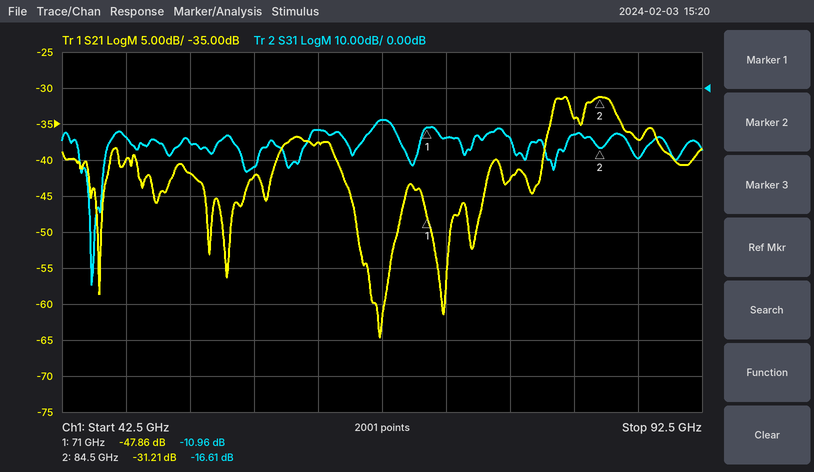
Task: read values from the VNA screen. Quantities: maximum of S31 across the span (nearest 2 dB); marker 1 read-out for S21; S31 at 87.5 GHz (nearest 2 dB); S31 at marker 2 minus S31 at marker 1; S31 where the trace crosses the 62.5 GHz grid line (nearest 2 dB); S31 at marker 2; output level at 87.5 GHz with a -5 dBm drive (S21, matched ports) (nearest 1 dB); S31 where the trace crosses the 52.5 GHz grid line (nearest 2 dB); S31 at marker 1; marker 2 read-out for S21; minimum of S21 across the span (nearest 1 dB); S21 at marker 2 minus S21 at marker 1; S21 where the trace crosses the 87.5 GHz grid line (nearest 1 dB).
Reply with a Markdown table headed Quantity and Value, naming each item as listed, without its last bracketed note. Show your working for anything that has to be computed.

| Quantity | Value |
|---|---|
| maximum of S31 across the span | -8 dB |
| marker 1 read-out for S21 | -47.86 dB |
| S31 at 87.5 GHz | -20 dB |
| S31 at marker 2 minus S31 at marker 1 | -16.61 − (-10.96) = -5.65 dB |
| S31 where the trace crosses the 62.5 GHz grid line | -12 dB |
| S31 at marker 2 | -16.61 dB |
| output level at 87.5 GHz with a -5 dBm drive (S21, matched ports) | -5 dBm + (-37 dB) = -42 dBm |
| S31 where the trace crosses the 52.5 GHz grid line | -16 dB |
| S31 at marker 1 | -10.96 dB |
| marker 2 read-out for S21 | -31.21 dB |
| minimum of S21 across the span | -65 dB |
| S21 at marker 2 minus S21 at marker 1 | -31.21 − (-47.86) = 16.65 dB |
| S21 where the trace crosses the 87.5 GHz grid line | -37 dB |
